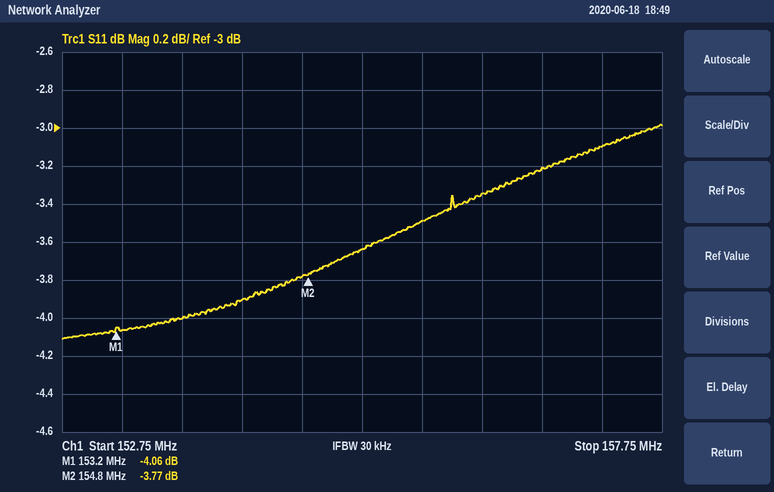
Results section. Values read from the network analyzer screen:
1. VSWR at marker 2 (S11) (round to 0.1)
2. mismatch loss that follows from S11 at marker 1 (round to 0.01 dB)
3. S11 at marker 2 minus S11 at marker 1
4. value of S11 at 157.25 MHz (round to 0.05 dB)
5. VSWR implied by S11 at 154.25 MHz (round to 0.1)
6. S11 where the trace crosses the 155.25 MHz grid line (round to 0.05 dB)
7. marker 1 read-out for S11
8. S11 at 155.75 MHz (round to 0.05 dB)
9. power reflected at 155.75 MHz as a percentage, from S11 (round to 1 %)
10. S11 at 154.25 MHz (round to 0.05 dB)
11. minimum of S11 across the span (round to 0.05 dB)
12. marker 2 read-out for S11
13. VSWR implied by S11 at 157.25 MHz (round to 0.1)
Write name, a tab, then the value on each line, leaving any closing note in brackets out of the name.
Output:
VSWR at marker 2 (S11)	4.7
mismatch loss that follows from S11 at marker 1	2.17 dB
S11 at marker 2 minus S11 at marker 1	0.29 dB
value of S11 at 157.25 MHz	-3.10 dB
VSWR implied by S11 at 154.25 MHz	4.5
S11 where the trace crosses the 155.25 MHz grid line	-3.65 dB
marker 1 read-out for S11	-4.06 dB
S11 at 155.75 MHz	-3.50 dB
power reflected at 155.75 MHz as a percentage, from S11	45 %
S11 at 154.25 MHz	-3.90 dB
minimum of S11 across the span	-4.10 dB
marker 2 read-out for S11	-3.77 dB
VSWR implied by S11 at 157.25 MHz	5.7
